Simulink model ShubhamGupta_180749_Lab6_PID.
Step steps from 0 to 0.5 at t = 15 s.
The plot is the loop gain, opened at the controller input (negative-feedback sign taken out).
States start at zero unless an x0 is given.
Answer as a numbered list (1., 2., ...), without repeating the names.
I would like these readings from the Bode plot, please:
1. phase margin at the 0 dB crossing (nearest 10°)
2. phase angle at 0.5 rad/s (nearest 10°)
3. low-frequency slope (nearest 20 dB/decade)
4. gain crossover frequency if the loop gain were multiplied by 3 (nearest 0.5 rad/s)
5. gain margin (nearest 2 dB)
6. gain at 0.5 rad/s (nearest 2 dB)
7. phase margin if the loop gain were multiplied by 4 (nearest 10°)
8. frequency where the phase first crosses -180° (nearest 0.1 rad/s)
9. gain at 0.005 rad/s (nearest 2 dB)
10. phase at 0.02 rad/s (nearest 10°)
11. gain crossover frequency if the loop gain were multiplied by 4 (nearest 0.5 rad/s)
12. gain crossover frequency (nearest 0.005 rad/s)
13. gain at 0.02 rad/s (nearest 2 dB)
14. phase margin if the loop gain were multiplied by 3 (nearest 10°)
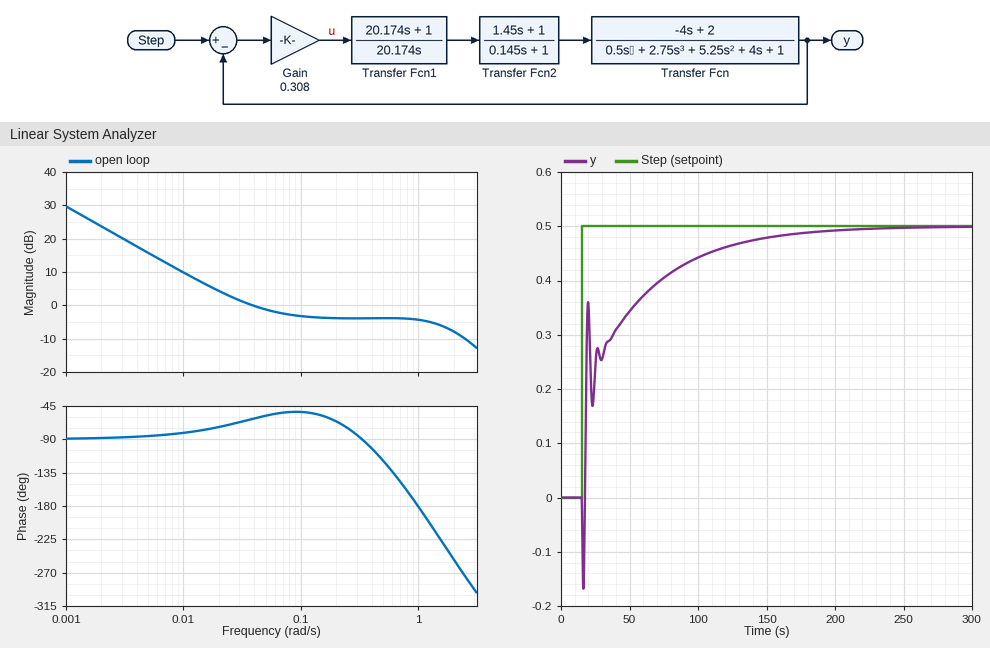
1. 120°
2. -120°
3. -20 dB/decade
4. 2.5 rad/s
5. 4 dB
6. -4 dB
7. -110°
8. 1.0 rad/s
9. 16 dB
10. -70°
11. 3.0 rad/s
12. 0.040 rad/s
13. 4 dB
14. -90°
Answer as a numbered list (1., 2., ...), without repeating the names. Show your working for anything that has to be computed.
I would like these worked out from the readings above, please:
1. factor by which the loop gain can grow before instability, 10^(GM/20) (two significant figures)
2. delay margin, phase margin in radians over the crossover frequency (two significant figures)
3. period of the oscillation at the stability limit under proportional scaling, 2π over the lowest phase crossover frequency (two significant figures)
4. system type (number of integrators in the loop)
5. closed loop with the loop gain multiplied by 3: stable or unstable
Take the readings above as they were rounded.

1. 10^(4 / 20) = 1.6
2. 120 × π / 180 / 0.04 = 52 s
3. 2π / 1 = 6.3 s
4. 1
5. unstable
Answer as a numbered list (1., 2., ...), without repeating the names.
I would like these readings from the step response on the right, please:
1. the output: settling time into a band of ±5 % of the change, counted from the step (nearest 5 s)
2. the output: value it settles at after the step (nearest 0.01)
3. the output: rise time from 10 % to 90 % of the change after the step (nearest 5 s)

1. 125 s
2. 0.50
3. 90 s
